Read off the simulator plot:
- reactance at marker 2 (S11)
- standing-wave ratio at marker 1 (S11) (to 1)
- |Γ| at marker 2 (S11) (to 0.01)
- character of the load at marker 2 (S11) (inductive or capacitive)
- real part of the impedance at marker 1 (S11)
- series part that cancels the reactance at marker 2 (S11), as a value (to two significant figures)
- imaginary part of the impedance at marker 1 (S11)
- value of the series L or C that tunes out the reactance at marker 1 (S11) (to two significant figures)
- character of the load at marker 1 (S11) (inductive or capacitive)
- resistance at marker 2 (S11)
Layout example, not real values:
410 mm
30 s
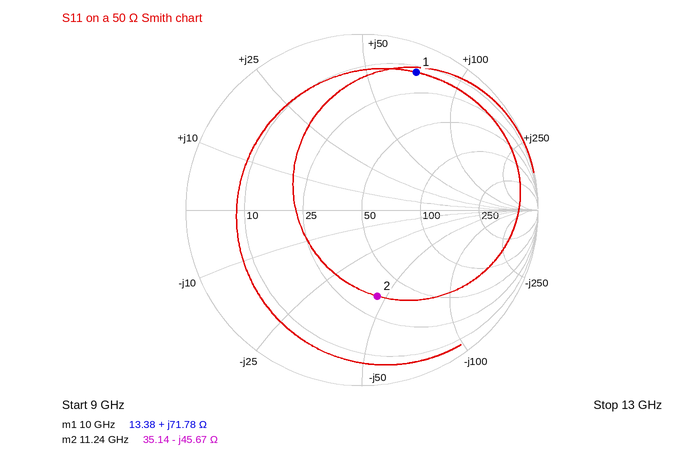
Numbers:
-45.67 Ω
12
0.50
capacitive
13.38 Ω
650 pH
+71.78 Ω
220 fF
inductive
35.14 Ω
